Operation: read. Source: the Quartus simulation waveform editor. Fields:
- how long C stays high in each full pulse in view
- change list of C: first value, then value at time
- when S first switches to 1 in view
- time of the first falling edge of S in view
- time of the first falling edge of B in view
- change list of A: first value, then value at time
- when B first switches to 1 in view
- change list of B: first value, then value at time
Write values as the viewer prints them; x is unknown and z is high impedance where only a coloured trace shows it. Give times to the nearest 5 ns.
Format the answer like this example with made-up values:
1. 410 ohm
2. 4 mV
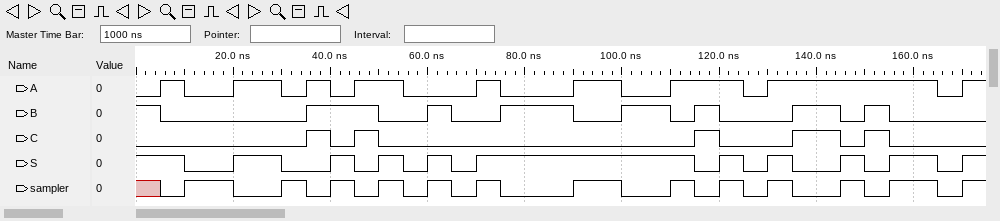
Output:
1. 5 ns, 5 ns, 5 ns, 10 ns, 5 ns
2. 0, 1 at 35 ns, 0 at 40 ns, 1 at 45 ns, 0 at 50 ns, 1 at 115 ns, 0 at 120 ns, 1 at 135 ns, 0 at 145 ns, 1 at 150 ns, 0 at 155 ns
3. 20 ns
4. 10 ns
5. 5 ns
6. 0, 1 at 5 ns, 0 at 10 ns, 1 at 20 ns, 0 at 30 ns, 1 at 35 ns, 0 at 40 ns, 1 at 45 ns, 0 at 55 ns, 1 at 70 ns, 0 at 75 ns, 1 at 90 ns, 0 at 100 ns, 1 at 110 ns, 0 at 125 ns, 1 at 130 ns, 0 at 165 ns, 1 at 170 ns
7. 35 ns
8. 1, 0 at 5 ns, 1 at 35 ns, 0 at 50 ns, 1 at 60 ns, 0 at 65 ns, 1 at 75 ns, 0 at 90 ns, 1 at 100 ns, 0 at 110 ns, 1 at 115 ns, 0 at 120 ns, 1 at 135 ns, 0 at 145 ns, 1 at 150 ns, 0 at 155 ns
